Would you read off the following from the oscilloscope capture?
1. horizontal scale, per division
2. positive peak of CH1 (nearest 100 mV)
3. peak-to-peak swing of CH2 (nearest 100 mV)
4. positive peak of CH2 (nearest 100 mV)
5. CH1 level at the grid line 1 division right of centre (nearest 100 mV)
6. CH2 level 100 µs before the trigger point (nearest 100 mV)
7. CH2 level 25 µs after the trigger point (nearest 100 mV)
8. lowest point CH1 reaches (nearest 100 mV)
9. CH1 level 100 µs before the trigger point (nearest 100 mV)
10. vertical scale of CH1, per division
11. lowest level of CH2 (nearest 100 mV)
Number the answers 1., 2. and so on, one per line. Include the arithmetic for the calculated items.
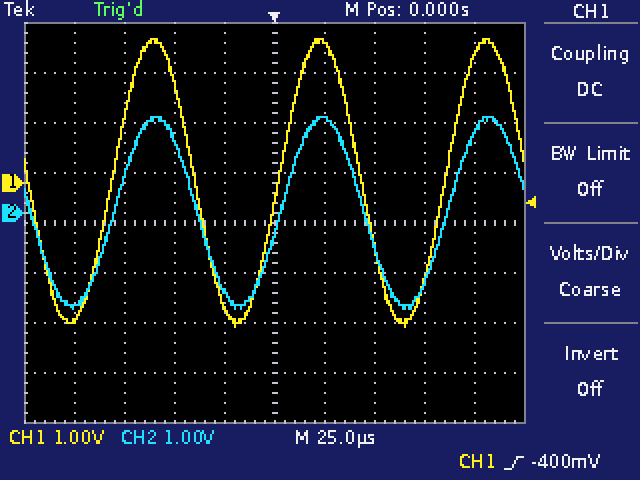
1. 25 µs
2. 2.9 V
3. 1.9 V − (-1.9 V) = 3.8 V
4. 1.9 V
5. 2.8 V
6. -1.9 V
7. 1.9 V
8. -2.9 V
9. -2.7 V
10. 1 V
11. -1.9 V
